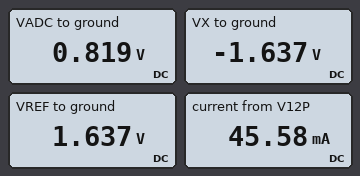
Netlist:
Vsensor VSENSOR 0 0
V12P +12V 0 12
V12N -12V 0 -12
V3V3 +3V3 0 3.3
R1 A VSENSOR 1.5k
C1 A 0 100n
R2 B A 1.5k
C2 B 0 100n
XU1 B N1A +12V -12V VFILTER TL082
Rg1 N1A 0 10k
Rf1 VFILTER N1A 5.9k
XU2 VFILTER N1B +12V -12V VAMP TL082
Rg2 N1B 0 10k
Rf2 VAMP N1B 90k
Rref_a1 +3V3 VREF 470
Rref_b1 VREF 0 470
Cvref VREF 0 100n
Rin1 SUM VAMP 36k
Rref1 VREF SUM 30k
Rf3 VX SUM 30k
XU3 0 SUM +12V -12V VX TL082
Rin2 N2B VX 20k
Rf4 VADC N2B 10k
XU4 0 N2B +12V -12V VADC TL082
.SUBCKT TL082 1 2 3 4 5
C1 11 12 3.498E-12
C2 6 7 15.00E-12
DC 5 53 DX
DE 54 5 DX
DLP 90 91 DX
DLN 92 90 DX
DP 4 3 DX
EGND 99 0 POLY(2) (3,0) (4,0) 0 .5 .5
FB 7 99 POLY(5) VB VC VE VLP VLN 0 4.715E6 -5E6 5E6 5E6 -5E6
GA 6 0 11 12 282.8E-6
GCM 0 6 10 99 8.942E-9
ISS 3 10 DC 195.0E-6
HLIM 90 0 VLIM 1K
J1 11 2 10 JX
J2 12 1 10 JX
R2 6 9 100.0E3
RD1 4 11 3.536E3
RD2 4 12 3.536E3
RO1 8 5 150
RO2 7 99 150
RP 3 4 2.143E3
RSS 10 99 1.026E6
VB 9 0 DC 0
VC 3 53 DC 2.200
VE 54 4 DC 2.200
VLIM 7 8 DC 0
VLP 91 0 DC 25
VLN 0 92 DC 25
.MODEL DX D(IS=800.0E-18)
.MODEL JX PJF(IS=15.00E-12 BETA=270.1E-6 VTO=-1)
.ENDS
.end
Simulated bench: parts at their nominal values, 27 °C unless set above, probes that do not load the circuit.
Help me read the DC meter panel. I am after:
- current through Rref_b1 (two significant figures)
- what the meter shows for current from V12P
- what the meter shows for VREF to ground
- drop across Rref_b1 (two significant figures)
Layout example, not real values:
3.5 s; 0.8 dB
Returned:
3.5 mA; 45.58 mA; 1.637 V; 1.6 V
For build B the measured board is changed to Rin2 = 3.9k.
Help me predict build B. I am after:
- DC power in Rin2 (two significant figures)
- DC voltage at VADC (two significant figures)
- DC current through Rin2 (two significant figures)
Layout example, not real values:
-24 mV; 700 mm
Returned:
690 µW; 4.2 V; 420 µA
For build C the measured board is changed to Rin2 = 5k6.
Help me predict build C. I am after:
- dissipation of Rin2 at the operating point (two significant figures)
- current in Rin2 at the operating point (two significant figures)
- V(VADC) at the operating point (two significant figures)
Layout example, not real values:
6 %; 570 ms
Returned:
480 µW; 290 µA; 2.9 V
